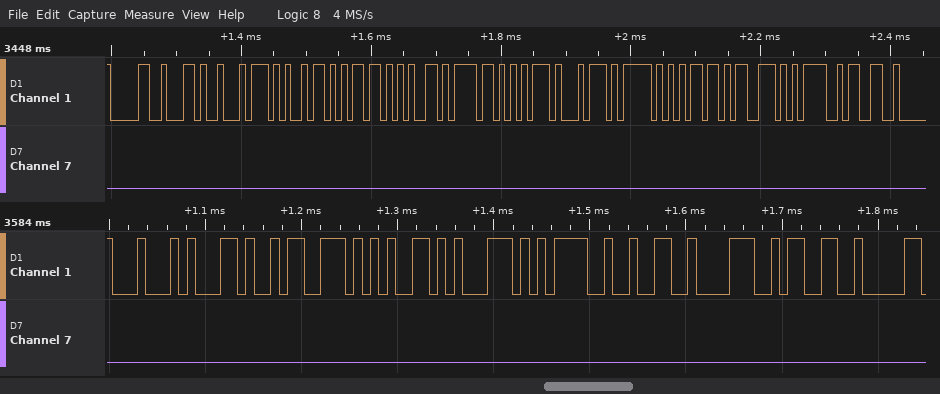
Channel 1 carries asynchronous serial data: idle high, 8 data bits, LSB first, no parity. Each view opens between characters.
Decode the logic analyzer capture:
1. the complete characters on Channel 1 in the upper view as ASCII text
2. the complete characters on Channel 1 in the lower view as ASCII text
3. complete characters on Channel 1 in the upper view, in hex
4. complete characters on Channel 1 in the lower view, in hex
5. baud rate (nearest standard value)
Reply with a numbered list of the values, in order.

1. "0,timeout_ms=3"
2. "D,seq=283"
3. 30, 2C, 74, 69, 6D, 65, 6F, 75, 74, 5F, 6D, 73, 3D, 33
4. 44, 2C, 73, 65, 71, 3D, 32, 38, 33
5. 115200 baud
